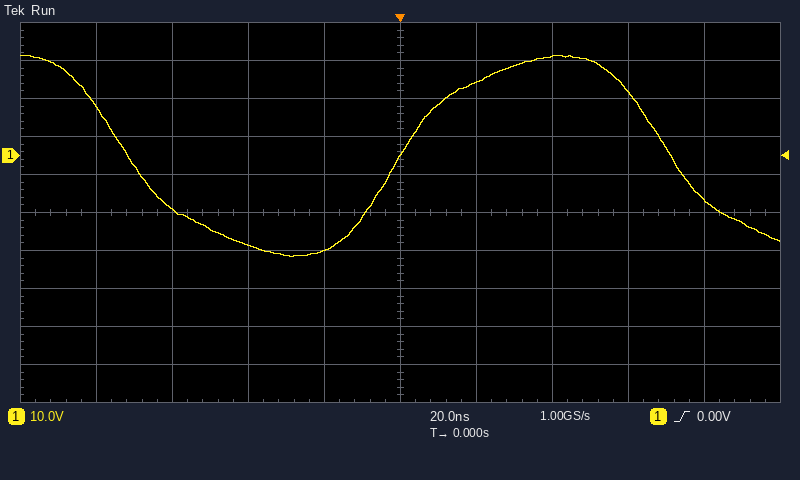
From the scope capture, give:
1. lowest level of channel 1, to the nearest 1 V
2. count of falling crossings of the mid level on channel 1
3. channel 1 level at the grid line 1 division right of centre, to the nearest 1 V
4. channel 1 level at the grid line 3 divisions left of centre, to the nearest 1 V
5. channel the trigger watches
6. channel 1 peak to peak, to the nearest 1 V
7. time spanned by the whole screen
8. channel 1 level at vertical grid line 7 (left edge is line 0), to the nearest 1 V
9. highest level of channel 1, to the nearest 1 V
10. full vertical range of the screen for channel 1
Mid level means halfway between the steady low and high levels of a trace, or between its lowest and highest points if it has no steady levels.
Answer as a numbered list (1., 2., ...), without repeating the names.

1. -27 V
2. 2
3. 19 V
4. -14 V
5. channel 1
6. 53 V
7. 200 ns
8. 26 V
9. 26 V
10. 100 V
